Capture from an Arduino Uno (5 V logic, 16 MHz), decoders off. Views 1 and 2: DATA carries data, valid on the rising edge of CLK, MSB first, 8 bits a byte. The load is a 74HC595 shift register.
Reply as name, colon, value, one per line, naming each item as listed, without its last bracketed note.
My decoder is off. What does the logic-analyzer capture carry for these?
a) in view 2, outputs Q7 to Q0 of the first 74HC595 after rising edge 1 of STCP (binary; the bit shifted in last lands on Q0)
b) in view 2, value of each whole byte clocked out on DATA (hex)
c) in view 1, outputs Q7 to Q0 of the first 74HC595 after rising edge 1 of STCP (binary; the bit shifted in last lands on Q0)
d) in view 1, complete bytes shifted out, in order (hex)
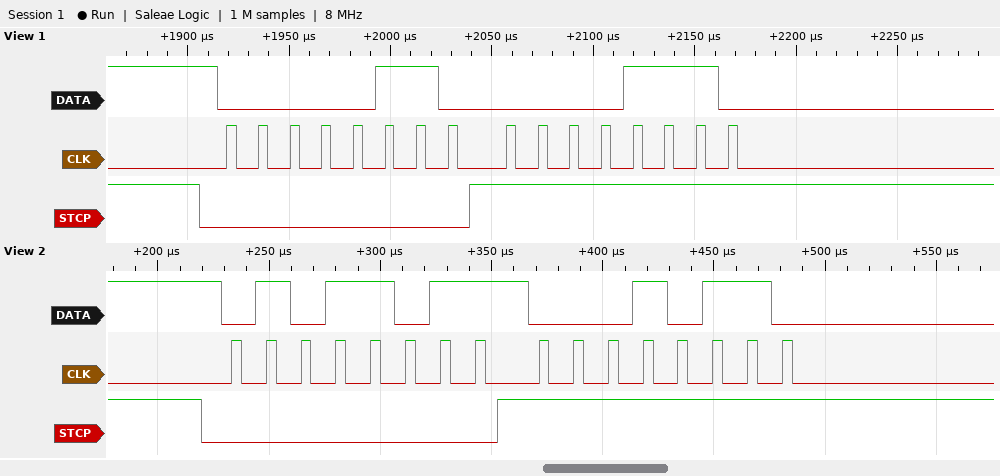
in view 2, outputs Q7 to Q0 of the first 74HC595 after rising edge 1 of STCP: 01011011
in view 2, value of each whole byte clocked out on DATA: 0x5B 0x16
in view 1, outputs Q7 to Q0 of the first 74HC595 after rising edge 1 of STCP: 00000110
in view 1, complete bytes shifted out, in order: 06 0E
